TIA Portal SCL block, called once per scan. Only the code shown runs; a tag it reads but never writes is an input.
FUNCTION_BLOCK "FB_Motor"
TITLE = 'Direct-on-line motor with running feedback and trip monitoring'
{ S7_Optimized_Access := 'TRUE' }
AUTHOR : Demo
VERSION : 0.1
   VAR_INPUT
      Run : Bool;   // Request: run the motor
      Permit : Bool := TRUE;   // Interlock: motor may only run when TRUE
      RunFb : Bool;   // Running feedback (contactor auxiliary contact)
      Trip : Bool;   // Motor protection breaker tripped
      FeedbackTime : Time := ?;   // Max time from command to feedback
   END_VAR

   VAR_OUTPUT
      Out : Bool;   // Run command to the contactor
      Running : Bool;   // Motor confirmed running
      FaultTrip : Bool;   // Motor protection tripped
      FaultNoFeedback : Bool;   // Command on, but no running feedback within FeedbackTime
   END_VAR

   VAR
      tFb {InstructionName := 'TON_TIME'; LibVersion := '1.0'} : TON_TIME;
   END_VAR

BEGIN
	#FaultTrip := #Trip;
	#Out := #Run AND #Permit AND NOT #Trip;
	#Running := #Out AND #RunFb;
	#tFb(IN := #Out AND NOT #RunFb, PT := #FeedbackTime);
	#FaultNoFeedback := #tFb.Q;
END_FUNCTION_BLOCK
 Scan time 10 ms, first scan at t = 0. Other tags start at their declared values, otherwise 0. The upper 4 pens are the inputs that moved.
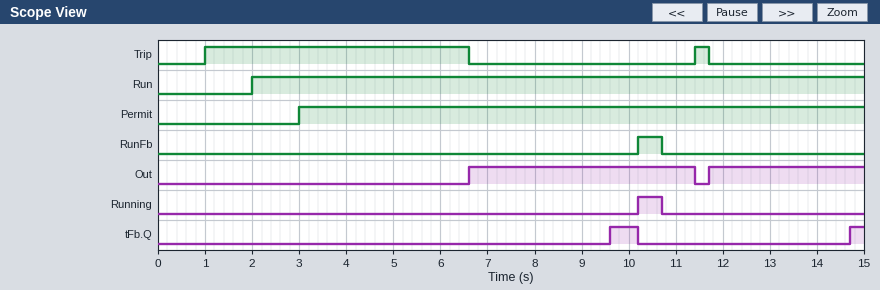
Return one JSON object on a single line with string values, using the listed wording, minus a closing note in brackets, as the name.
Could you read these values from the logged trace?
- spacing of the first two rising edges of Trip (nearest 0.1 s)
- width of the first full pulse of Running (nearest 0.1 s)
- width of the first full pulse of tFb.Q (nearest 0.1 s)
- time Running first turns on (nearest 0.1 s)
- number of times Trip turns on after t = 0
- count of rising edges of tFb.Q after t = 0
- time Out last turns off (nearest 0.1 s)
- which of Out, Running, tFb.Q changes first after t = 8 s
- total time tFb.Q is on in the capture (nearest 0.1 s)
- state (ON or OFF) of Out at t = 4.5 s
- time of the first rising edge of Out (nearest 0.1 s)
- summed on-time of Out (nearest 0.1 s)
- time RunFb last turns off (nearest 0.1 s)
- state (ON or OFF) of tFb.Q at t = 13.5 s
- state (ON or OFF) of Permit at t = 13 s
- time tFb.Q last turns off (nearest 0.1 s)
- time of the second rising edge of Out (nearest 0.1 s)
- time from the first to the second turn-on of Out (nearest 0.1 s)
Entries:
{"spacing of the first two rising edges of Trip": "10.4 s", "width of the first full pulse of Running": "0.5 s", "width of the first full pulse of tFb.Q": "0.6 s", "time Running first turns on": "10.2 s", "number of times Trip turns on after t = 0": "2", "count of rising edges of tFb.Q after t = 0": "2", "time Out last turns off": "11.4 s", "which of Out, Running, tFb.Q changes first after t = 8 s": "tFb.Q", "total time tFb.Q is on in the capture": "0.9 s", "state (ON or OFF) of Out at t = 4.5 s": "OFF", "time of the first rising edge of Out": "6.6 s", "summed on-time of Out": "8.1 s", "time RunFb last turns off": "10.7 s", "state (ON or OFF) of tFb.Q at t = 13.5 s": "OFF", "state (ON or OFF) of Permit at t = 13 s": "ON", "time tFb.Q last turns off": "10.2 s", "time of the second rising edge of Out": "11.7 s", "time from the first to the second turn-on of Out": "5.1 s"}
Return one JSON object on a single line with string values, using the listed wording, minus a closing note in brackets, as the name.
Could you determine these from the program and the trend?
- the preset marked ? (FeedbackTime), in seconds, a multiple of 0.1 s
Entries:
{"the preset marked ? (FeedbackTime), in seconds, a multiple of 0.1 s": "3.0 s"}
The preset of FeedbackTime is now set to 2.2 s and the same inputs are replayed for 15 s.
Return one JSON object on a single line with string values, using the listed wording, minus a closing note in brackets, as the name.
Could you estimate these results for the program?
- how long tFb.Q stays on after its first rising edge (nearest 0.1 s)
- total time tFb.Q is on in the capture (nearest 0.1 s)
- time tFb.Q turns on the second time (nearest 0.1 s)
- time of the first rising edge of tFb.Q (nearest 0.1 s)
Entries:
{"how long tFb.Q stays on after its first rising edge": "1.4 s", "total time tFb.Q is on in the capture": "2.5 s", "time tFb.Q turns on the second time": "13.9 s", "time of the first rising edge of tFb.Q": "8.8 s"}
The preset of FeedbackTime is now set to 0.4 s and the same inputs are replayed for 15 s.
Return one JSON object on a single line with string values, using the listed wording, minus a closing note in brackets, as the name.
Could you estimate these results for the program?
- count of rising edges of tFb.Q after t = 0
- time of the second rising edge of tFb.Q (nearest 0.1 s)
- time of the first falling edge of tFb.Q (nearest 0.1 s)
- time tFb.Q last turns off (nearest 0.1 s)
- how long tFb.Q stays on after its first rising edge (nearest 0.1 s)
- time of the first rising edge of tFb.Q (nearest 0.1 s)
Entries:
{"count of rising edges of tFb.Q after t = 0": "3", "time of the second rising edge of tFb.Q": "11.1 s", "time of the first falling edge of tFb.Q": "10.2 s", "time tFb.Q last turns off": "11.4 s", "how long tFb.Q stays on after its first rising edge": "3.2 s", "time of the first rising edge of tFb.Q": "7.0 s"}
